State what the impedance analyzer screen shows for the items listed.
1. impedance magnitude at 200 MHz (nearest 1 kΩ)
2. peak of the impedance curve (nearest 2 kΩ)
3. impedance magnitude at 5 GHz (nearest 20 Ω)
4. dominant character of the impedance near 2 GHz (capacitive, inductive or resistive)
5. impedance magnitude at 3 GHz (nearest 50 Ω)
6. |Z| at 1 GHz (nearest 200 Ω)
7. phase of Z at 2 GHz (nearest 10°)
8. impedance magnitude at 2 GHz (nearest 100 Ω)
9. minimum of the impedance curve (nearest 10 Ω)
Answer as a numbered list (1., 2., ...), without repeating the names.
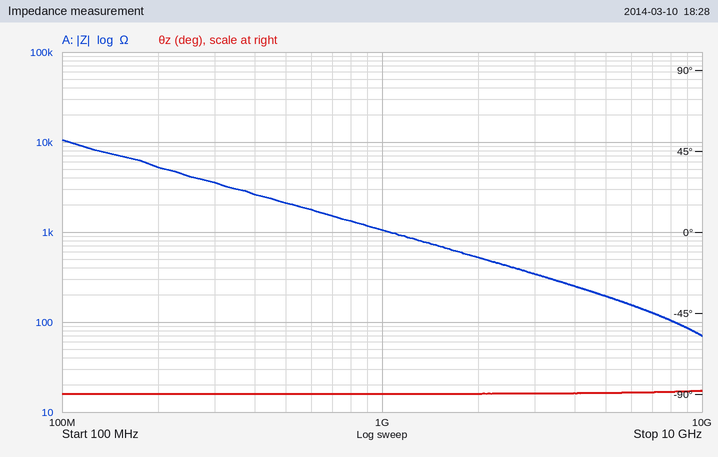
1. 5 kΩ
2. 10 kΩ
3. 200 Ω
4. capacitive
5. 350 Ω
6. 1.0 kΩ
7. -90°
8. 500 Ω
9. 70 Ω
